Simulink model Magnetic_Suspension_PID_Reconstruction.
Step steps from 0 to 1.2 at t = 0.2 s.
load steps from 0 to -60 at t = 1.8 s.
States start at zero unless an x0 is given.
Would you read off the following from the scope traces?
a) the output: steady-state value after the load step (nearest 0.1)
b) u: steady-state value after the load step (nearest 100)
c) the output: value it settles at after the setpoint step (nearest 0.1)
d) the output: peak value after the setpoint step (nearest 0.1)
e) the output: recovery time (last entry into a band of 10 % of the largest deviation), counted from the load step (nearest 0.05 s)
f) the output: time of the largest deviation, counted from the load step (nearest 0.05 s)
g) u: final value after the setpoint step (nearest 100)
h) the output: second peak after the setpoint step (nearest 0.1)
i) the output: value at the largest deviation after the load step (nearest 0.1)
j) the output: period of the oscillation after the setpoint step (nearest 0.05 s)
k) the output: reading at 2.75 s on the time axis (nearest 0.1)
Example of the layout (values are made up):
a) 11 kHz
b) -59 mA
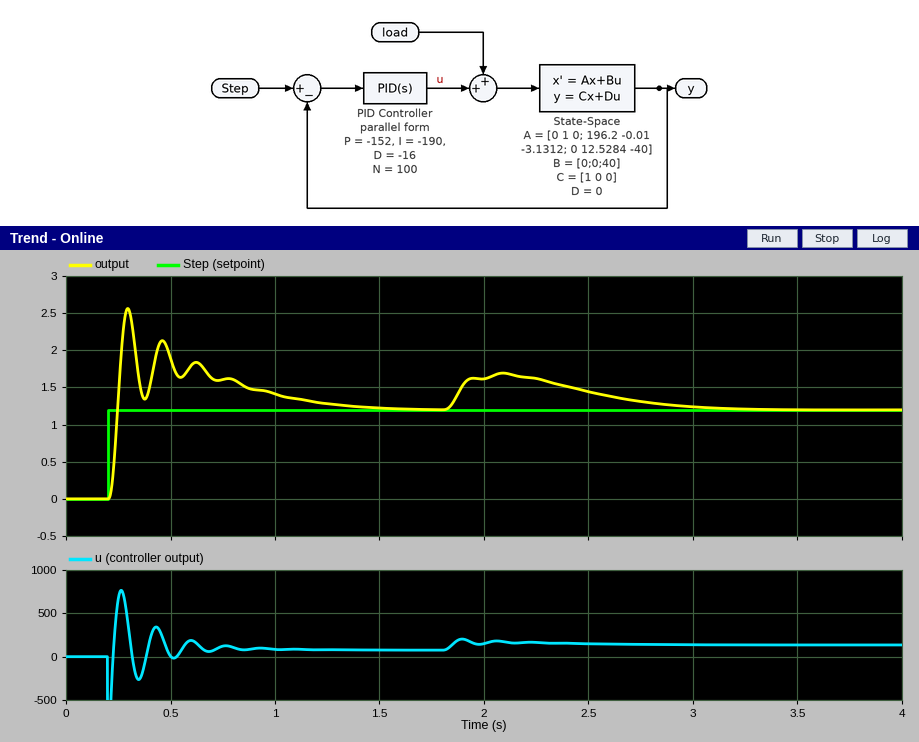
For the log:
a) 1.2
b) 100
c) 1.2
d) 2.6
e) 1.15 s
f) 0.30 s
g) 100
h) 2.1
i) 1.7
j) 0.15 s
k) 1.3
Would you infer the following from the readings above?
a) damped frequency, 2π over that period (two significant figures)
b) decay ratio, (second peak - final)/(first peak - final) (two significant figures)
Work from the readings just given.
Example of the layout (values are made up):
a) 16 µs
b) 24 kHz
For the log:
a) 42 rad/s
b) 0.64
